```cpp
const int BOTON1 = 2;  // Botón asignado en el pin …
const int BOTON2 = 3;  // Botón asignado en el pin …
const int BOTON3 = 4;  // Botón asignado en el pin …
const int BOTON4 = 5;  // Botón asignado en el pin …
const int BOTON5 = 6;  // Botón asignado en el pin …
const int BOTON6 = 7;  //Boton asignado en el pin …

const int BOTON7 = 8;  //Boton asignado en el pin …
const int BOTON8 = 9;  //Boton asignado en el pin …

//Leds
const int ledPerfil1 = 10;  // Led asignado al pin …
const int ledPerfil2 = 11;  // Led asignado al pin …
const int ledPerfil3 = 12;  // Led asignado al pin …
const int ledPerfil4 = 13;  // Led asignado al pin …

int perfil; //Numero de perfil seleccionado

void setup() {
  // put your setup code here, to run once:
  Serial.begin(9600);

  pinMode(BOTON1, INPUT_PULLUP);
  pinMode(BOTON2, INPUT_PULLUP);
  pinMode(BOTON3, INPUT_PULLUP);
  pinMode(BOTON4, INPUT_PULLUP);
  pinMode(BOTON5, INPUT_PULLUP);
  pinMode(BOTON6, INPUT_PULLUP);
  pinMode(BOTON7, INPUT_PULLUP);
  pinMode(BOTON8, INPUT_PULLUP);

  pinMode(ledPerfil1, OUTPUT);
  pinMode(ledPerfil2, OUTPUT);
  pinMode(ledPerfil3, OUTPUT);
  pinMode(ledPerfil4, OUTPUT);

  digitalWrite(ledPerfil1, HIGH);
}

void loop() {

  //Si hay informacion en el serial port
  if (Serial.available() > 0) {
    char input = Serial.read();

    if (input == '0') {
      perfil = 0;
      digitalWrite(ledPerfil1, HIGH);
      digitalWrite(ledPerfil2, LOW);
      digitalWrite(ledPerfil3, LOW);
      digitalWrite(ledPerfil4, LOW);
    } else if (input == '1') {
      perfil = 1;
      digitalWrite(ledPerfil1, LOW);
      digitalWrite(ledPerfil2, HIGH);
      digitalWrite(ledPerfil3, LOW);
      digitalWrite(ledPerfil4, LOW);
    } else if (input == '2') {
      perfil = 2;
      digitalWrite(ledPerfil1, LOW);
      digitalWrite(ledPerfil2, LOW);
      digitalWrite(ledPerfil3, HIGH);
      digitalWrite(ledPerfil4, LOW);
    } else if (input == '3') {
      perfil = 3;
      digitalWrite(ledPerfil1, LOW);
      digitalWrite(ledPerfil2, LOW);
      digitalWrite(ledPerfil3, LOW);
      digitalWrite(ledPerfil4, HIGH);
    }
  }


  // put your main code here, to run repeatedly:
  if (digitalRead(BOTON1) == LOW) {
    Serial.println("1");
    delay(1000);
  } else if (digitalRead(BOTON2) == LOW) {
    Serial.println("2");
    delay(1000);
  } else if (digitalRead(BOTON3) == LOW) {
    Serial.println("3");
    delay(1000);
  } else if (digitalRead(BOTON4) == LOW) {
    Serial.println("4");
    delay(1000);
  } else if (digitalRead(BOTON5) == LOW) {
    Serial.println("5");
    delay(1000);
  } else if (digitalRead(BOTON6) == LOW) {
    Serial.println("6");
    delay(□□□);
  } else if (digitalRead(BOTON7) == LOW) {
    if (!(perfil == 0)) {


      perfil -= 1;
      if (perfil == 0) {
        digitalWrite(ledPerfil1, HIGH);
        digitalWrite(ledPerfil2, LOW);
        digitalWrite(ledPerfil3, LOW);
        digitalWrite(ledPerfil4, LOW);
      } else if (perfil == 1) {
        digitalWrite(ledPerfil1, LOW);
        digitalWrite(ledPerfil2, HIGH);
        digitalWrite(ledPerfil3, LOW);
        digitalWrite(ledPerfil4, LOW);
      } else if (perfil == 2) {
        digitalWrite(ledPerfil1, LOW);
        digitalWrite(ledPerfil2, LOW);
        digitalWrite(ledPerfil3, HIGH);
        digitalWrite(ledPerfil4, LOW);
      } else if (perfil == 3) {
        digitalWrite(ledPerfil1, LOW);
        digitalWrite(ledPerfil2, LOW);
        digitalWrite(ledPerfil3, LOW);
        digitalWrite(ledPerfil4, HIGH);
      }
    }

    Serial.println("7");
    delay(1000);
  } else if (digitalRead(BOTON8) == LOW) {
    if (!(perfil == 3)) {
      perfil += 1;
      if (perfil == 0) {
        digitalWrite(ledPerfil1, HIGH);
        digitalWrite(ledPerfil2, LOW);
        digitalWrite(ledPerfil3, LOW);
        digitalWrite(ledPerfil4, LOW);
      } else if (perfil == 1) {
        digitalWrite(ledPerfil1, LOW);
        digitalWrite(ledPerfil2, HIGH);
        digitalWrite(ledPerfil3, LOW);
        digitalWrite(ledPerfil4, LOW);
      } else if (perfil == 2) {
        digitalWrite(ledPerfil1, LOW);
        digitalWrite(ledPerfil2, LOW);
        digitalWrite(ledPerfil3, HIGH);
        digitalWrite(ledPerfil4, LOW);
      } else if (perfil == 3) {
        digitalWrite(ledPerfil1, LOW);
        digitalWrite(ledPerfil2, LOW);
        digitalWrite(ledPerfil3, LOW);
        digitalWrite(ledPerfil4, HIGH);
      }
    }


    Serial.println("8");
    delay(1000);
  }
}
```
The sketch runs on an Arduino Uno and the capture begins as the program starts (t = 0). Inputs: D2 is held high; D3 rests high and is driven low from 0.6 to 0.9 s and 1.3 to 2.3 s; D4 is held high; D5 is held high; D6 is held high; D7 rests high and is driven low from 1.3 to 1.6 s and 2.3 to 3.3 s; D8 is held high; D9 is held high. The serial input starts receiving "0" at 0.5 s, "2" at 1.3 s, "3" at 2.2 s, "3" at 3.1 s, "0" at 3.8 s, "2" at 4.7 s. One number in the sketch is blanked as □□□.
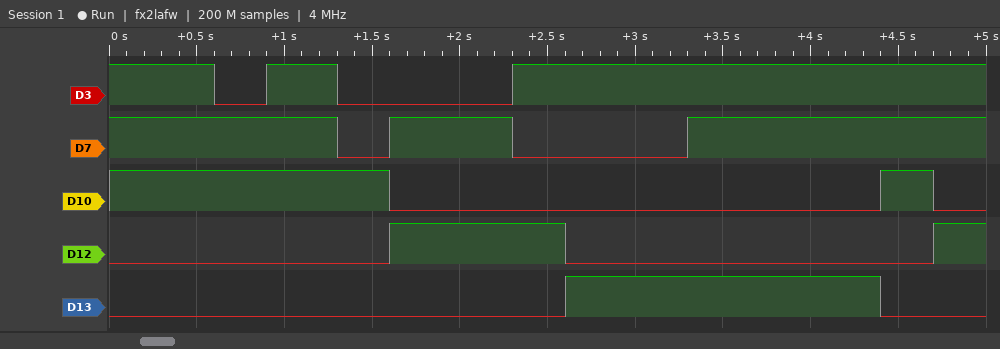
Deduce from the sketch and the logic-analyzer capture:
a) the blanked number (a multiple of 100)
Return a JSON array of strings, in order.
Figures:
["1800"]
